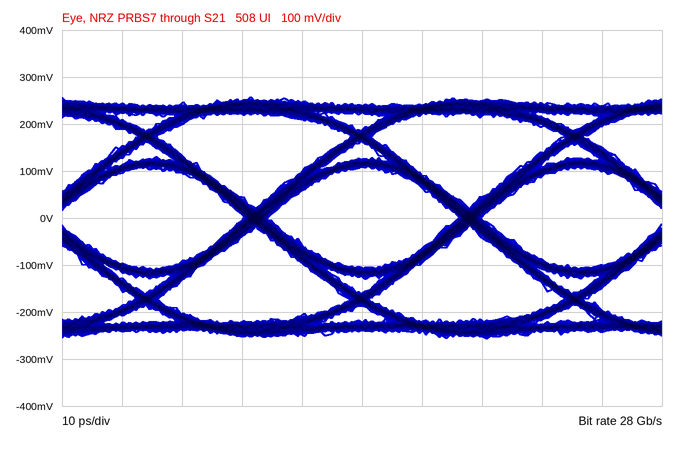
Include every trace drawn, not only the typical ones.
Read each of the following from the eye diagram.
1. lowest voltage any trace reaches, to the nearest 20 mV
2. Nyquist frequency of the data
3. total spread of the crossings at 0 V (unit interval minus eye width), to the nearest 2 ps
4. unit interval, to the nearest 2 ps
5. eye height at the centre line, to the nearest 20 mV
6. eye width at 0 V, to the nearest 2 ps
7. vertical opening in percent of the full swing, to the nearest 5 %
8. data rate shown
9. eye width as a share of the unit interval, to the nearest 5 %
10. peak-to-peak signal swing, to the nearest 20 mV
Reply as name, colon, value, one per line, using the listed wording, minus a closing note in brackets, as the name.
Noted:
lowest voltage any trace reaches, to the nearest 20 mV: -260 mV
Nyquist frequency of the data: 14 GHz
total spread of the crossings at 0 V (unit interval minus eye width), to the nearest 2 ps: 4 ps
unit interval, to the nearest 2 ps: 36 ps
eye height at the centre line, to the nearest 20 mV: 220 mV
eye width at 0 V, to the nearest 2 ps: 32 ps
vertical opening in percent of the full swing, to the nearest 5 %: 40 %
data rate shown: 28 Gb/s
eye width as a share of the unit interval, to the nearest 5 %: 90 %
peak-to-peak signal swing, to the nearest 20 mV: 520 mV
